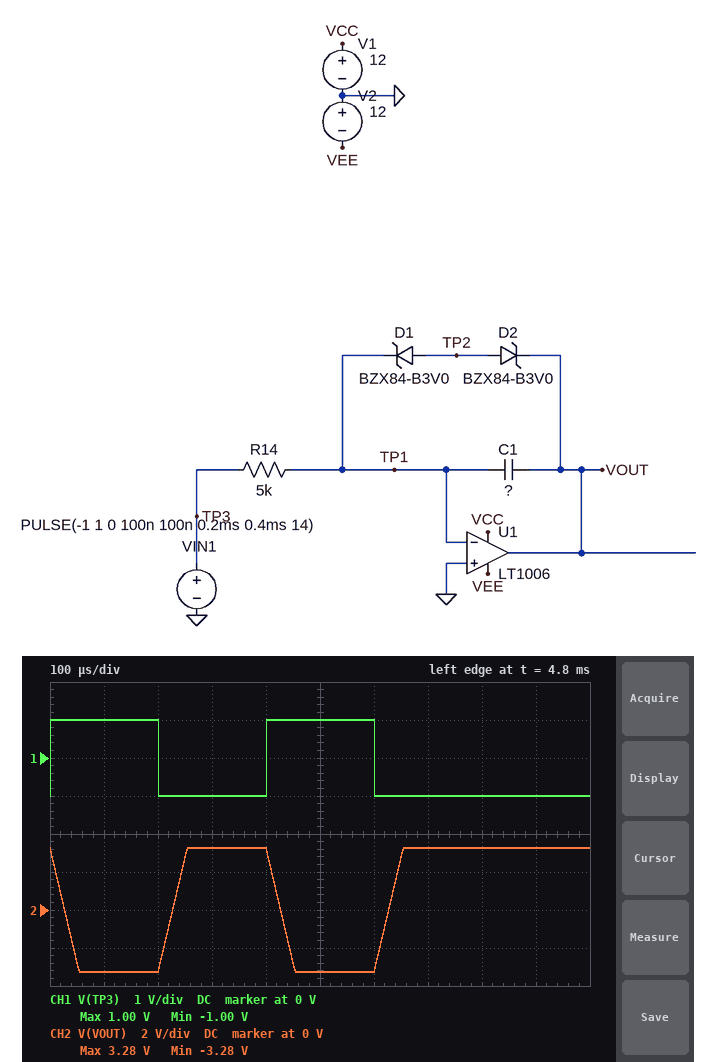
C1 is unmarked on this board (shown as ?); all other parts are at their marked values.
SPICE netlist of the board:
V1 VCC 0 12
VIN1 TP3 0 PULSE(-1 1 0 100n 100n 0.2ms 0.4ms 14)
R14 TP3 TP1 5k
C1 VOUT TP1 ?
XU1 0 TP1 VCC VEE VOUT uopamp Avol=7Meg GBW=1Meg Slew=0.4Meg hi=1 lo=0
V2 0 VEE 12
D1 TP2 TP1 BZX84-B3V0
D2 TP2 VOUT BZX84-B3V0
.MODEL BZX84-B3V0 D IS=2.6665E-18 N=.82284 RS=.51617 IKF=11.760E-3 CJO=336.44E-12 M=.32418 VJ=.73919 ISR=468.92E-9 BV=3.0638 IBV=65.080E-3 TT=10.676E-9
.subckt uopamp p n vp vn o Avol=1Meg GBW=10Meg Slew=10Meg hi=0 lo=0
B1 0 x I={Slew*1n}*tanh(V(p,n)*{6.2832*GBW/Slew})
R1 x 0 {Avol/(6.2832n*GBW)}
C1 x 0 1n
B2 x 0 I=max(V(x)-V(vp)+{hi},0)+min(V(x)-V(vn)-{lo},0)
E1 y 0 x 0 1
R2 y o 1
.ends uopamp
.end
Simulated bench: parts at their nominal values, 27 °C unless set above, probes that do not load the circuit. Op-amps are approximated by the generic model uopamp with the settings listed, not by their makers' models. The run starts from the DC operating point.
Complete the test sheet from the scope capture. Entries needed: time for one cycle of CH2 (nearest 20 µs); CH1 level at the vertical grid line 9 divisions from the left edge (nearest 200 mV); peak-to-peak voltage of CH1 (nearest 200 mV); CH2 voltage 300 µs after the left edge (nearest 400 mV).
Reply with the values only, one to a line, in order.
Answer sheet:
400 µs
-1.0 V
2.0 V
3.2 V
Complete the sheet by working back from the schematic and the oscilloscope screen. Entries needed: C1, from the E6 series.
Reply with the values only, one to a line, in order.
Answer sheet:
1.5 nF
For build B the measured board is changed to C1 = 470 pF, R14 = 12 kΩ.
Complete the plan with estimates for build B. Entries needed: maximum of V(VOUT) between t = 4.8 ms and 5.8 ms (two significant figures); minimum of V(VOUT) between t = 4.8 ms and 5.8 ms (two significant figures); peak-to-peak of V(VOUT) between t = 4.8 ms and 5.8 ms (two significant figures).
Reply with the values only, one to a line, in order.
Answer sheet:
3.2 V
-3.2 V
6.4 V
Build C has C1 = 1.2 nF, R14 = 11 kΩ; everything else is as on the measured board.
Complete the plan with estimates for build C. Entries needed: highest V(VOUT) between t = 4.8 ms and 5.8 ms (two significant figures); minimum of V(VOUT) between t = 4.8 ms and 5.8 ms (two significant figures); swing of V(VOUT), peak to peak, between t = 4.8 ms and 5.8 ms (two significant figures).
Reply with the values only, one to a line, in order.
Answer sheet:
3.2 V
-3.2 V
6.4 V
